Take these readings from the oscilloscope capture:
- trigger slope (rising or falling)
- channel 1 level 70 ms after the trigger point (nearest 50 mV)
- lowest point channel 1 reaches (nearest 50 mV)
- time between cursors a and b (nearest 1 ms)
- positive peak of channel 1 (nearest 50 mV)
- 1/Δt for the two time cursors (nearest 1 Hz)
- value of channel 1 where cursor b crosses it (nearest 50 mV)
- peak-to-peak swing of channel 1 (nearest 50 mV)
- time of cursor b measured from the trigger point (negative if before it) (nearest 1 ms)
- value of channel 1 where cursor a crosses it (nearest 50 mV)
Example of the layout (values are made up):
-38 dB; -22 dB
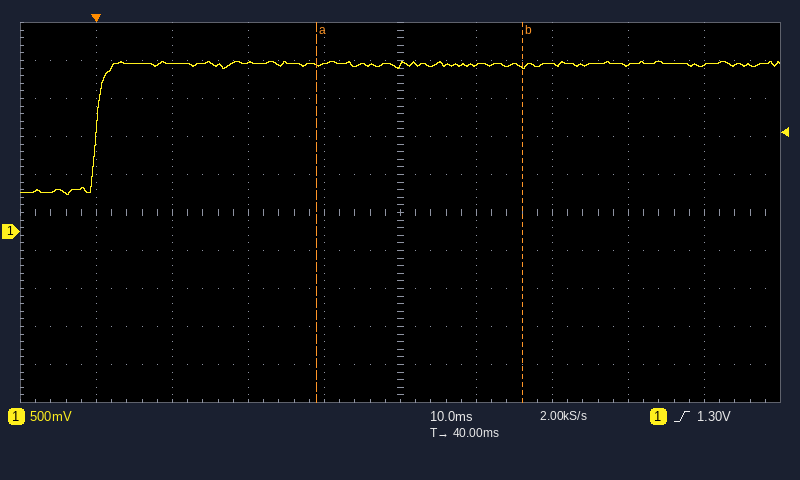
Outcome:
rising; 2.20 V; 500 mV; 27 ms; 2.25 V; 37 Hz; 2.15 V; 1.75 V; +56 ms; 2.20 V
